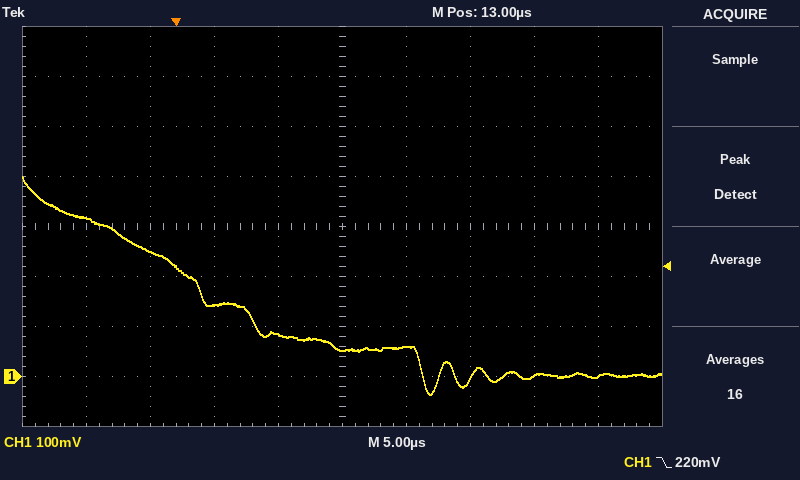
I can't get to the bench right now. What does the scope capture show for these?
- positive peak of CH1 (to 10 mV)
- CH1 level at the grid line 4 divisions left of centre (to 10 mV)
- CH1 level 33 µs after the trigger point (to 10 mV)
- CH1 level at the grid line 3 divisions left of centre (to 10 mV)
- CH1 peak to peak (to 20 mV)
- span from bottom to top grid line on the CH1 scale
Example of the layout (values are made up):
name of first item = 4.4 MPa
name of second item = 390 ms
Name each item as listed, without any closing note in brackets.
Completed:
positive peak of CH1 = 400 mV
CH1 level at the grid line 4 divisions left of centre = 320 mV
CH1 level 33 µs after the trigger point = 0 mV
CH1 level at the grid line 3 divisions left of centre = 250 mV
CH1 peak to peak = 440 mV
span from bottom to top grid line on the CH1 scale = 800 mV
